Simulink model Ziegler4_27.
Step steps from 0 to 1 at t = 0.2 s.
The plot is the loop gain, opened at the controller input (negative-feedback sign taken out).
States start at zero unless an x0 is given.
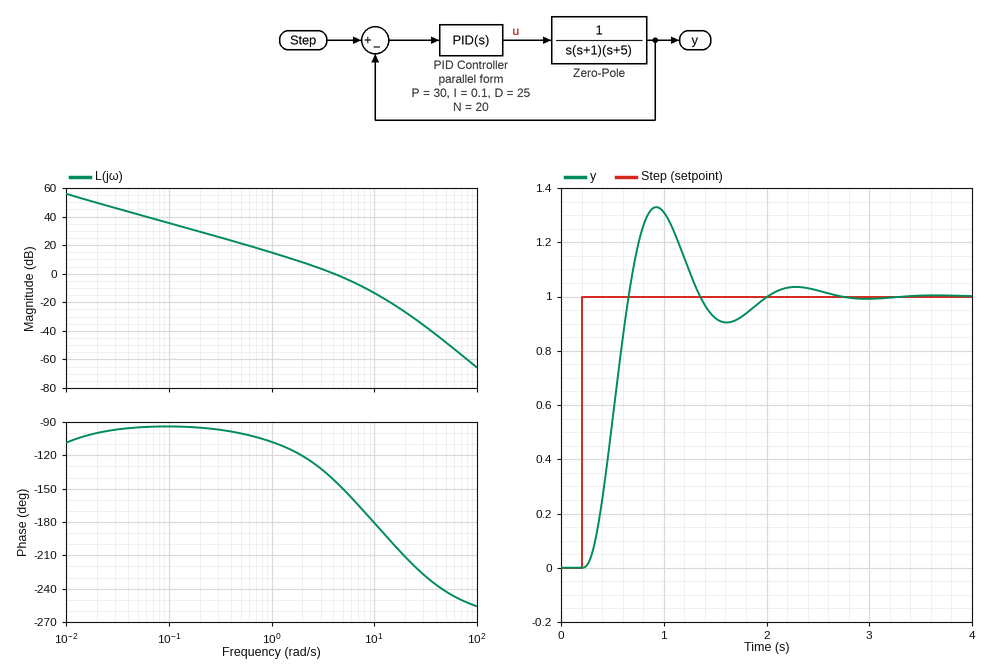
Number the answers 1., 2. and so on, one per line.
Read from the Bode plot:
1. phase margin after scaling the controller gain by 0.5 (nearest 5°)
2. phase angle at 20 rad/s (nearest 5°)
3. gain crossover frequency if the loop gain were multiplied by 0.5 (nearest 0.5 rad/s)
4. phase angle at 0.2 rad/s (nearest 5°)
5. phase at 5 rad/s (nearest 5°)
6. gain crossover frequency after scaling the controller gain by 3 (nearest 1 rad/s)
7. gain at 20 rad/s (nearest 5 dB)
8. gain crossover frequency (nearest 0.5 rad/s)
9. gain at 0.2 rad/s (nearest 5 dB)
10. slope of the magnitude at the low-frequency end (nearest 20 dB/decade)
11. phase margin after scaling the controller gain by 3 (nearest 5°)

1. 55°
2. -210°
3. 2.5 rad/s
4. -95°
5. -150°
6. 8 rad/s
7. -25 dB
8. 4.0 rad/s
9. 30 dB
10. -20 dB/decade
11. 10°
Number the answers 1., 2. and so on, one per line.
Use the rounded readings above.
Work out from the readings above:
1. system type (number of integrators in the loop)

1. 1
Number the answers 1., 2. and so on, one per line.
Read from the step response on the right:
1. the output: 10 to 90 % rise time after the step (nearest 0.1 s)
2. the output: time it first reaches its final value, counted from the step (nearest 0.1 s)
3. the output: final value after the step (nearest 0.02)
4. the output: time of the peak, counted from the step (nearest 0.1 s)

1. 0.3 s
2. 0.5 s
3. 1.00
4. 0.7 s
